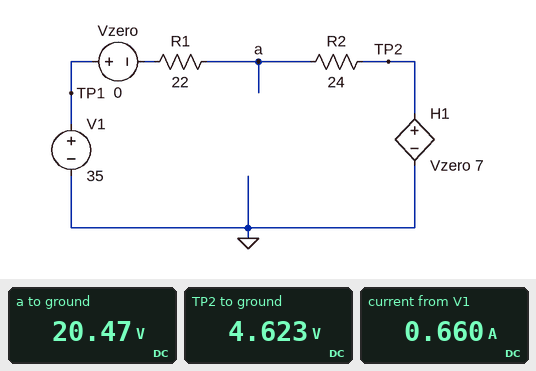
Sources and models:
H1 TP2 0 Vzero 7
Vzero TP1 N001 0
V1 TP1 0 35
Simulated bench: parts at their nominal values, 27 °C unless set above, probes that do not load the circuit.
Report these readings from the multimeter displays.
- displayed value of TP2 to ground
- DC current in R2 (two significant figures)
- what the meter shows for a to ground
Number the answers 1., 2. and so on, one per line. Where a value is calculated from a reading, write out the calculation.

1. 4.623 V
2. (20.47 V - 4.623 V) / 24 Ω = 660 mA
3. 20.47 V
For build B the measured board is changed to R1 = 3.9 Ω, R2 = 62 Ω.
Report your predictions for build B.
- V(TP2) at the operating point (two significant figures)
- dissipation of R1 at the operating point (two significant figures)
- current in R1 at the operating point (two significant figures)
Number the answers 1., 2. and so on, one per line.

1. 3.4 V
2. 900 mW
3. 480 mA
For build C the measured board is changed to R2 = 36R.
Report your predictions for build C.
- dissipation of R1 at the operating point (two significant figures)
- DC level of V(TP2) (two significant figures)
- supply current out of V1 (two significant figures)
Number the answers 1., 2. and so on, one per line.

1. 6.4 W
2. 3.8 V
3. 540 mA
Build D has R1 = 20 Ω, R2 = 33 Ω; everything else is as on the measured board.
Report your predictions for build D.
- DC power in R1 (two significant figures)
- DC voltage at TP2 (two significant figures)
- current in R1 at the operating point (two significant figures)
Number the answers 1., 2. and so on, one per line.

1. 6.8 W
2. 4.1 V
3. 580 mA
